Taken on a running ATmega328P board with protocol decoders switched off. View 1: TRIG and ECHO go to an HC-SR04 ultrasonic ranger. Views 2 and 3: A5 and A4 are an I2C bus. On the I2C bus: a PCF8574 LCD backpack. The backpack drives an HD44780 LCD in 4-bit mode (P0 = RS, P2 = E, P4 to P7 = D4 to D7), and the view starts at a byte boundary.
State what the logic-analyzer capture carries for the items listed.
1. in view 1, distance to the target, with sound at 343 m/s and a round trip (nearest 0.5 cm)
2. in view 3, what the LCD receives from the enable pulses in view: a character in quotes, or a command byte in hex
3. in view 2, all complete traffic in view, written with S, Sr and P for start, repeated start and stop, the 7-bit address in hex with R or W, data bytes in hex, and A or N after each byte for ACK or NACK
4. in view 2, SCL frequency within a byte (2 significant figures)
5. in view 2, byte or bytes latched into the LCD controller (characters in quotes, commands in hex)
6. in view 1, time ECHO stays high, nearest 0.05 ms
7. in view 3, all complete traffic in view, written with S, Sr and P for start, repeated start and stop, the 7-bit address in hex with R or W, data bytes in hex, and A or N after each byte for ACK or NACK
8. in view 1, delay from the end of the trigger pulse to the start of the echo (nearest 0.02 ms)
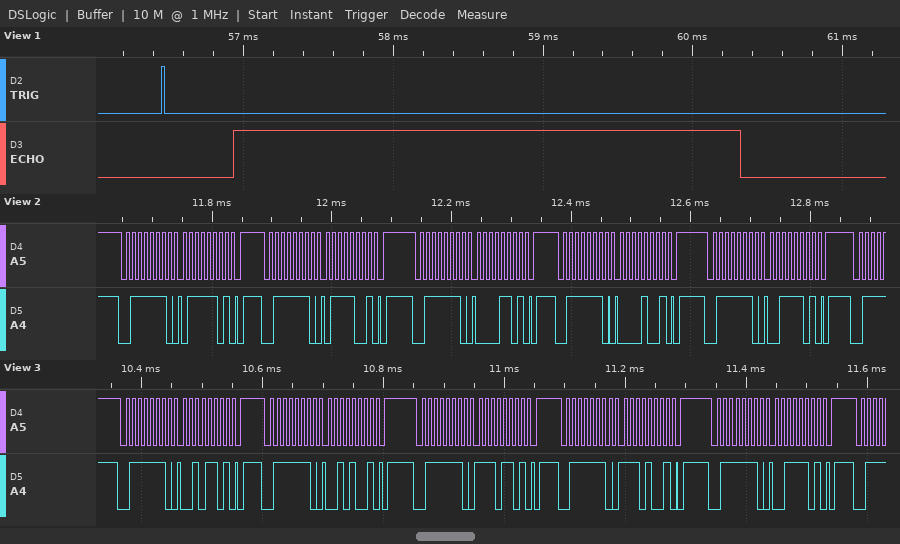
58 cm
'.'
S 3FW A 7D A P S 3FW A 79 A P S 3FW A 0D A P S 3FW A 09 A P S 3FW A 3D A P
100 kHz
'p'
3.40 ms
S 3FW A 2D A P S 3FW A 29 A P S 3FW A ED A P S 3FW A E9 A P S 3FW A 3D A P
0.46 ms
